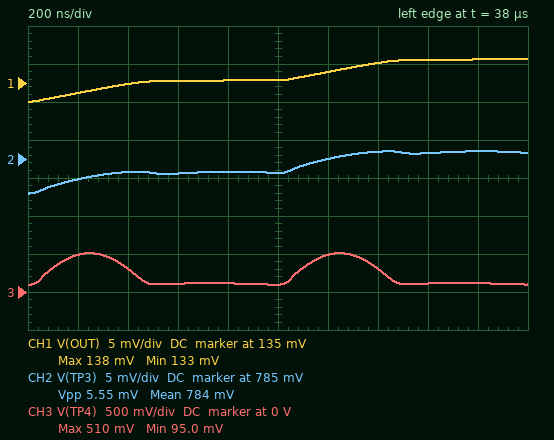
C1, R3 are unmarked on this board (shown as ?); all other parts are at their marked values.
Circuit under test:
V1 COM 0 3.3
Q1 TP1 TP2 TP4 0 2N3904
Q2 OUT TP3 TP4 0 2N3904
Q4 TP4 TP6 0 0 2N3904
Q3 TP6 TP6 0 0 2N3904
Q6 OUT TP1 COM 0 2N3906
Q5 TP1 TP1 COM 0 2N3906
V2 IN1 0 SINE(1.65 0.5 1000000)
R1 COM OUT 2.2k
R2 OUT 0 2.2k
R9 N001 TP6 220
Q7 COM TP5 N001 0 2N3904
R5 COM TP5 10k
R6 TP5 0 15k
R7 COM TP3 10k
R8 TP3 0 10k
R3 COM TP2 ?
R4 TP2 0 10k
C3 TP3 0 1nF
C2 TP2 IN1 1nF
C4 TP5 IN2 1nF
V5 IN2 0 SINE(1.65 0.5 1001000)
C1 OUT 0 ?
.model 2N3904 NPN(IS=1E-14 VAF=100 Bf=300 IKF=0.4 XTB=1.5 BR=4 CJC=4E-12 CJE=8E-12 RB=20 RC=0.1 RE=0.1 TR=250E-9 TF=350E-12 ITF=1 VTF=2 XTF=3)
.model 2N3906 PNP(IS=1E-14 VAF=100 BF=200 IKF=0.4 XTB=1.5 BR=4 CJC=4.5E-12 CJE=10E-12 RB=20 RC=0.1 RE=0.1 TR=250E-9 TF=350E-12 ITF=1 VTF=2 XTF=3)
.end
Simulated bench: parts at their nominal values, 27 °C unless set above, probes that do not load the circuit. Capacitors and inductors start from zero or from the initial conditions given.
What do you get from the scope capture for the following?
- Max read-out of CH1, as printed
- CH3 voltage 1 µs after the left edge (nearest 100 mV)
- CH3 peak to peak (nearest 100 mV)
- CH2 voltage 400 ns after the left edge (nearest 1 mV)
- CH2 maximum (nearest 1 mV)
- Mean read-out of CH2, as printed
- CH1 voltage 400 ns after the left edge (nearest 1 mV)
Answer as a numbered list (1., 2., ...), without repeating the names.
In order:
1. 138 mV
2. 100 mV
3. 400 mV
4. 783 mV
5. 786 mV
6. 784 mV
7. 135 mV
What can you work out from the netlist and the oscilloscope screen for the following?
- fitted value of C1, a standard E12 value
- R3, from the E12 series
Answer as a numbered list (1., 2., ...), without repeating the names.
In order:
1. 1.2 µF
2. 33 kΩ
